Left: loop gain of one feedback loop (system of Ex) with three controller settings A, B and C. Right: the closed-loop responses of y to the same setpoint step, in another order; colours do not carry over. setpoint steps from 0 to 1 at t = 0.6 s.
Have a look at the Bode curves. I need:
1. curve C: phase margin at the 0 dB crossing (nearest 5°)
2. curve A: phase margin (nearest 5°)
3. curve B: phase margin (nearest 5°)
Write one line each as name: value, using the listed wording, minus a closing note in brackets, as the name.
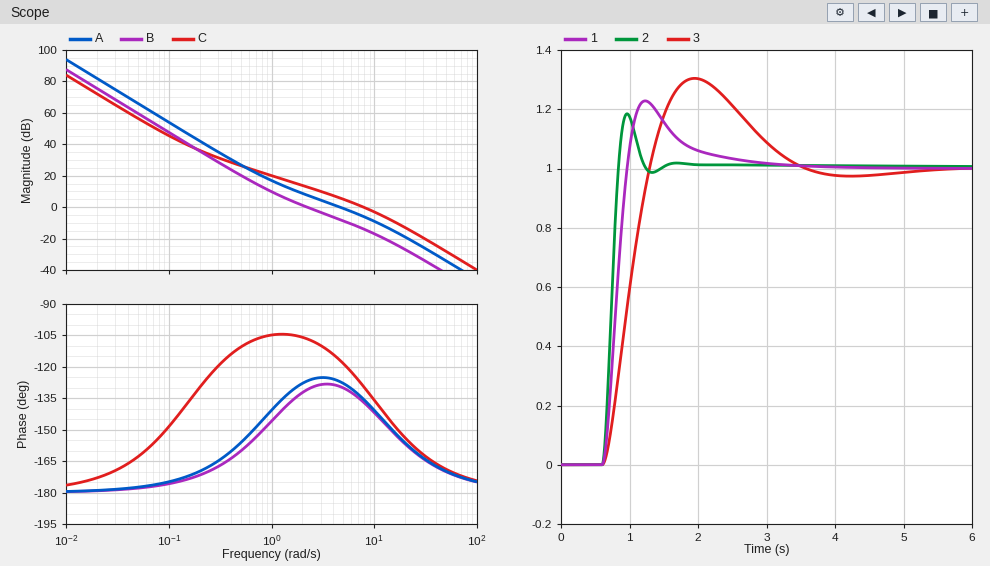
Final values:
curve C: phase margin at the 0 dB crossing: 50°
curve A: phase margin: 55°
curve B: phase margin: 50°
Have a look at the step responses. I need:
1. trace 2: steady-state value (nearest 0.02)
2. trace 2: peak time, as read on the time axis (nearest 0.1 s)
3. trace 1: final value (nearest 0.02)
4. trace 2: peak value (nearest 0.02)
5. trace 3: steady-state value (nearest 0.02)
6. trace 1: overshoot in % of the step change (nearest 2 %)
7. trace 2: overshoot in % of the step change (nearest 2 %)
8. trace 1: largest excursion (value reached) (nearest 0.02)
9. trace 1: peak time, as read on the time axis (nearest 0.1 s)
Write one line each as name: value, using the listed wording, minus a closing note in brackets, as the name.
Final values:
trace 2: steady-state value: 1.00
trace 2: peak time, as read on the time axis: 1.0 s
trace 1: final value: 1.00
trace 2: peak value: 1.18
trace 3: steady-state value: 1.00
trace 1: overshoot in % of the step change: 22 %
trace 2: overshoot in % of the step change: 18 %
trace 1: largest excursion (value reached): 1.22
trace 1: peak time, as read on the time axis: 1.2 s
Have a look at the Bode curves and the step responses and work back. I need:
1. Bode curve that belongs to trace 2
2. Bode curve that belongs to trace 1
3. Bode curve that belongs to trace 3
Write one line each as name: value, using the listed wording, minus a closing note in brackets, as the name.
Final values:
Bode curve that belongs to trace 2: C
Bode curve that belongs to trace 1: A
Bode curve that belongs to trace 3: B
